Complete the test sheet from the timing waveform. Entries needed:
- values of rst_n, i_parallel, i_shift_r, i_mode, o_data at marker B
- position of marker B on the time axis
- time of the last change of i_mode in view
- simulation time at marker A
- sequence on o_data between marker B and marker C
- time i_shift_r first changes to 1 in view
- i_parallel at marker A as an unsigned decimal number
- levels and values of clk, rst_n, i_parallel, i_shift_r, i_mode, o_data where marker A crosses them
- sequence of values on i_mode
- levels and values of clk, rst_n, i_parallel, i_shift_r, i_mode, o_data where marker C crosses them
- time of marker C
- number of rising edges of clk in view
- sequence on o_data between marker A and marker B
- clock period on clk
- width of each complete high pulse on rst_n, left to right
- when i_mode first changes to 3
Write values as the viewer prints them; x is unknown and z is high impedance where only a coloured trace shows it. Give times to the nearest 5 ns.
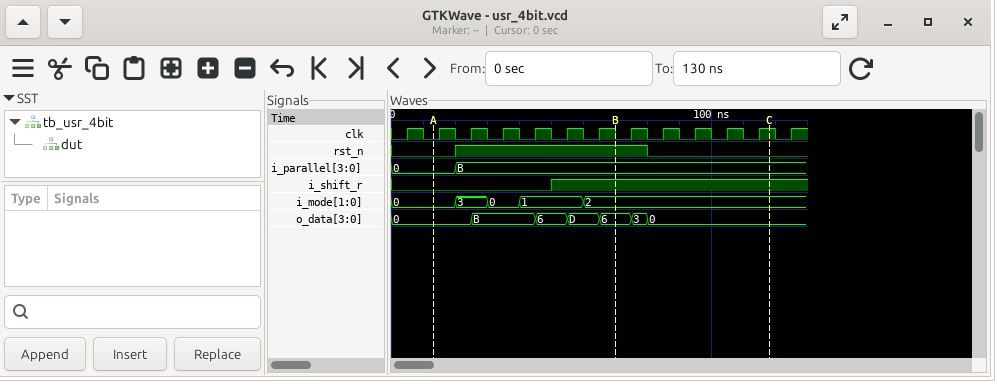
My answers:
rst_n=1, i_parallel=B, i_shift_r=1, i_mode=2, o_data=6
70 ns
60 ns
15 ns
6, 3, 0
50 ns
0
clk=0, rst_n=0, i_parallel=0, i_shift_r=0, i_mode=0, o_data=0
0, 3, 0, 1, 2
clk=1, rst_n=0, i_parallel=B, i_shift_r=1, i_mode=2, o_data=0
120 ns
13
0, B, 6, D, 6
10 ns
60 ns
20 ns
